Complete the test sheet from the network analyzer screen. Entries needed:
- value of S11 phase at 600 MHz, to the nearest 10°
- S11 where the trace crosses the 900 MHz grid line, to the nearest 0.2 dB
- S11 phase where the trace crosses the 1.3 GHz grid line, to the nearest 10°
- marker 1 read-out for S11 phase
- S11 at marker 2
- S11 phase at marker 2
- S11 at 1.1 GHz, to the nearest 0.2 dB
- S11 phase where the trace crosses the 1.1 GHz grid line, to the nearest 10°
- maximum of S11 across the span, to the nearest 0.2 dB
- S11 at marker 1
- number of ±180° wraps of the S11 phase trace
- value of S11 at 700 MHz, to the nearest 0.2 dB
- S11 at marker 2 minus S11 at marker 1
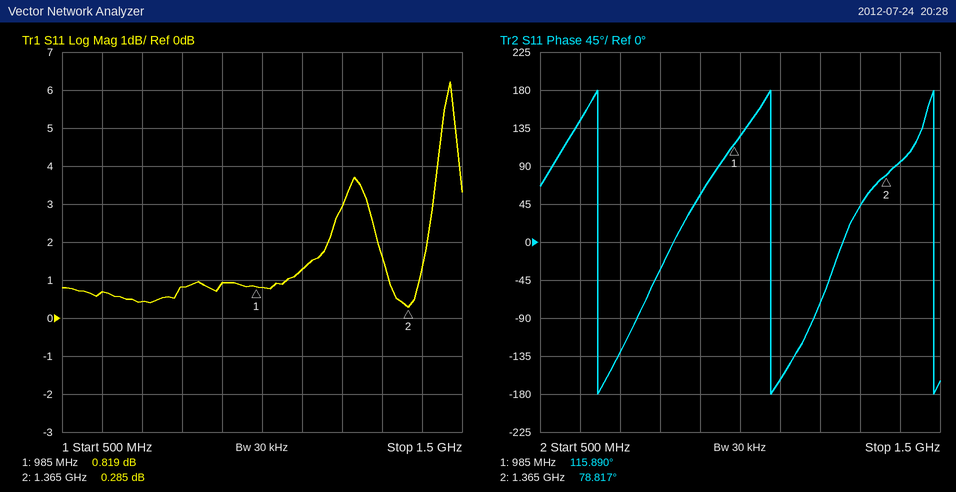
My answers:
140°
1.0 dB
40°
115.890°
0.285 dB
78.817°
1.2 dB
-160°
6.2 dB
0.819 dB
3
0.4 dB
-0.534 dB
